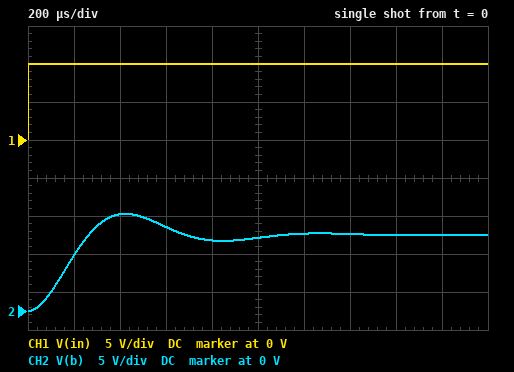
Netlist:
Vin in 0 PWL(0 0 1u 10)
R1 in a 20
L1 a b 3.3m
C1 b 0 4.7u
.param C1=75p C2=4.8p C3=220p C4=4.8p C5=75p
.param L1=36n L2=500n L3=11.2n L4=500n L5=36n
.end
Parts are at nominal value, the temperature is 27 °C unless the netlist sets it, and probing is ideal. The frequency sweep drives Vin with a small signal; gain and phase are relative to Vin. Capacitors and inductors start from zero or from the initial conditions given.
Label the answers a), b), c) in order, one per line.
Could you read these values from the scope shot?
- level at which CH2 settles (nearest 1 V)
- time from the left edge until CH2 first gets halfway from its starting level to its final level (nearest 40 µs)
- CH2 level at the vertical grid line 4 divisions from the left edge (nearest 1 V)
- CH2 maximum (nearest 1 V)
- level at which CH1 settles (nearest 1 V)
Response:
a) 10 V
b) 160 µs
c) 9 V
d) 13 V
e) 10 V
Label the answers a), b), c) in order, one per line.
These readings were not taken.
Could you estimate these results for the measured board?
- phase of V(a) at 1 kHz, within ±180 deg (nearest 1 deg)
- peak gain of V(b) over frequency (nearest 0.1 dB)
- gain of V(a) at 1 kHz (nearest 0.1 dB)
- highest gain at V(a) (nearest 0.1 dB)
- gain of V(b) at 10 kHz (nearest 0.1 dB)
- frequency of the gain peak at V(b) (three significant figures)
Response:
a) -57 deg
b) 3.1 dB
c) -5.2 dB
d) 0 dB
e) -35.6 dB
f) 1.08 kHz
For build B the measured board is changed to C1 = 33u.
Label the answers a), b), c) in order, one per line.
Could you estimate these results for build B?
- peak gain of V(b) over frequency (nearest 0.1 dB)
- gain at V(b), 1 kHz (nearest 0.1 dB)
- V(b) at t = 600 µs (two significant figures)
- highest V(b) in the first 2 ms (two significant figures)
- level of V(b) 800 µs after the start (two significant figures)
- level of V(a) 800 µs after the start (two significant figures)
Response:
a) 0 dB
b) -14.5 dB
c) 5.4 V
d) 9.8 V
e) 7.0 V
f) 5.7 V
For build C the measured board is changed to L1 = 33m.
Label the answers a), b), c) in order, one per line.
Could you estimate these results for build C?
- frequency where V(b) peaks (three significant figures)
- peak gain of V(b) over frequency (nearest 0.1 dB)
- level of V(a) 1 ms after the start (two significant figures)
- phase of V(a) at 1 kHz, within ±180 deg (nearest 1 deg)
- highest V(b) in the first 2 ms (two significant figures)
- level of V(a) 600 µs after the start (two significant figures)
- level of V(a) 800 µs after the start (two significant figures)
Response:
a) 398 Hz
b) 12.5 dB
c) 9.0 V
d) 7 deg
e) 17 V
f) 8.0 V
g) 8.3 V
